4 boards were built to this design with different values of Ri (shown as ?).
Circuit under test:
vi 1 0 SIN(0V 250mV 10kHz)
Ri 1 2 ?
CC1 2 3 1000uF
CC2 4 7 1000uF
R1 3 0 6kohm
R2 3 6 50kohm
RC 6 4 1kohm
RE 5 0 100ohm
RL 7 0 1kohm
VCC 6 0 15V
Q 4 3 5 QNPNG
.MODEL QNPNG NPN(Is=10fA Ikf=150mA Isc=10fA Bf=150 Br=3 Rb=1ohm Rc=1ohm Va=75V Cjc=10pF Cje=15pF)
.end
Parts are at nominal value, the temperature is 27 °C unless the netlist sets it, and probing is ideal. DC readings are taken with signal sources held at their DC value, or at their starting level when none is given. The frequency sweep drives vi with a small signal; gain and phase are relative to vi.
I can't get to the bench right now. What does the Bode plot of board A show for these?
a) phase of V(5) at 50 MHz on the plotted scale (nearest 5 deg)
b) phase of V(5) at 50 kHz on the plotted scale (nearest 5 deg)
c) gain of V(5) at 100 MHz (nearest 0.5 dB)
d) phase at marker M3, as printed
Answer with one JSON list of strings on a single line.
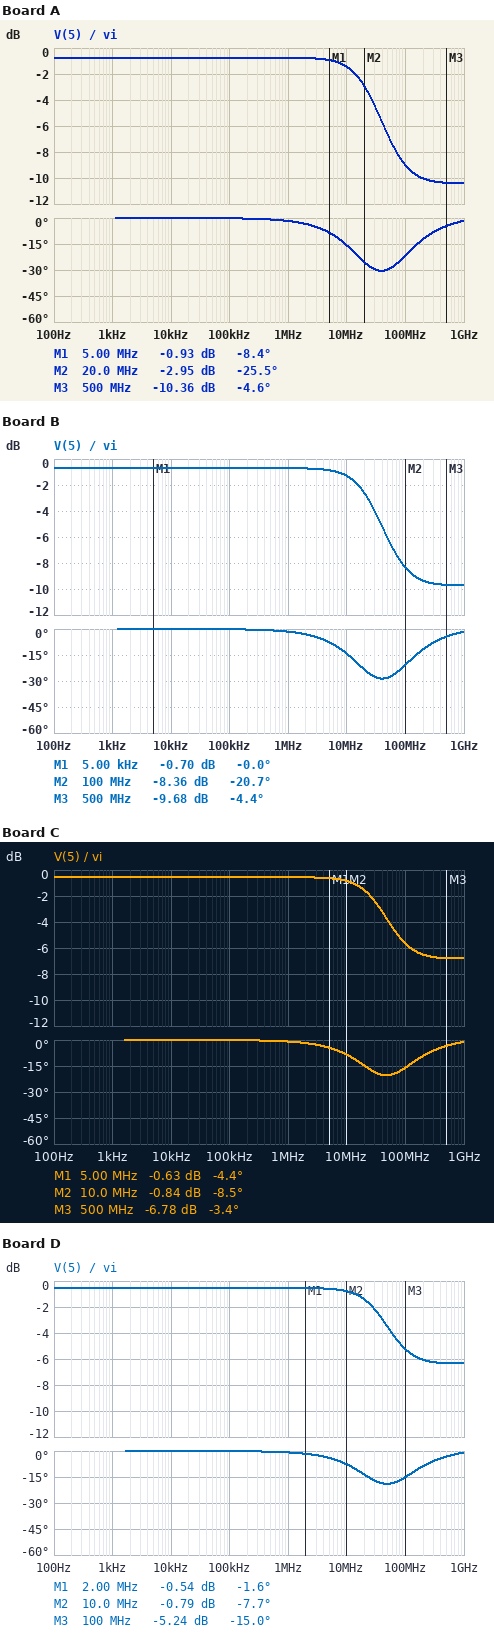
["-30 deg", "0 deg", "-9.0 dB", "-4.6 deg"]
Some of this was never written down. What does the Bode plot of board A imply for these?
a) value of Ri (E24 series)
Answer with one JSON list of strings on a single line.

["180 Ω"]
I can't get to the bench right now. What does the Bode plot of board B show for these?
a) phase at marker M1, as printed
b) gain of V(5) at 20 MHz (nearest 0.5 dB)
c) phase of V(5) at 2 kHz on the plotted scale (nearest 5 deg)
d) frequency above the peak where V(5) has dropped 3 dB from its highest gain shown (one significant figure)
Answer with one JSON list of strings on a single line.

["-0.0 deg", "-2.5 dB", "0 deg", "30 MHz"]
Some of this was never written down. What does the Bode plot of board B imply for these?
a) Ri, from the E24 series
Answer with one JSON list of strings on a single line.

["160 Ω"]
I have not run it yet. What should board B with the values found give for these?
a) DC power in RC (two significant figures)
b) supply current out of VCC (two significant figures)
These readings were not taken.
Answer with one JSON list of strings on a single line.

["45 mW", "7.0 mA"]
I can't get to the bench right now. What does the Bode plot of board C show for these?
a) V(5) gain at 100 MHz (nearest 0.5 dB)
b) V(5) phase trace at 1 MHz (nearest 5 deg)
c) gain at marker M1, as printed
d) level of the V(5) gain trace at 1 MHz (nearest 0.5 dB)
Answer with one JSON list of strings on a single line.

["-5.5 dB", "0 deg", "-0.63 dB", "-0.5 dB"]
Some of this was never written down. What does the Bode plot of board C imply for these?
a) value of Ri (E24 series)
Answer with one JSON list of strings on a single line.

["91 Ω"]
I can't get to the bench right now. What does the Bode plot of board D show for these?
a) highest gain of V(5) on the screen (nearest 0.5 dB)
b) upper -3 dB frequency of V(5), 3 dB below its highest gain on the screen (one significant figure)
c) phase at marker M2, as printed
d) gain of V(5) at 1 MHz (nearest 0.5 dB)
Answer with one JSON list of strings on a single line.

["-0.5 dB", "50 MHz", "-7.7 deg", "-0.5 dB"]
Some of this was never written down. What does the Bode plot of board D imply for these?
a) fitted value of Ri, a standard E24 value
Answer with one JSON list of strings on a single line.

["82 Ω"]
